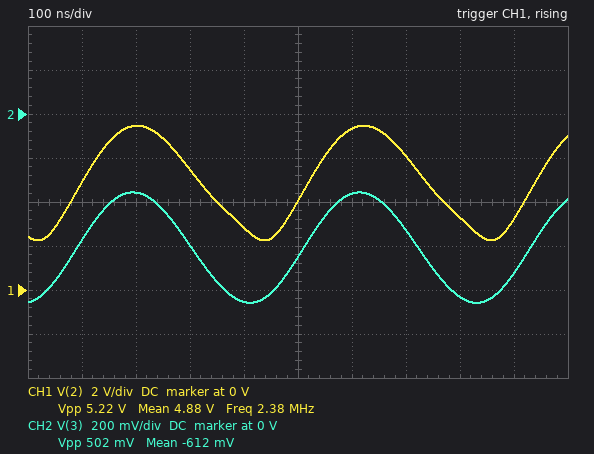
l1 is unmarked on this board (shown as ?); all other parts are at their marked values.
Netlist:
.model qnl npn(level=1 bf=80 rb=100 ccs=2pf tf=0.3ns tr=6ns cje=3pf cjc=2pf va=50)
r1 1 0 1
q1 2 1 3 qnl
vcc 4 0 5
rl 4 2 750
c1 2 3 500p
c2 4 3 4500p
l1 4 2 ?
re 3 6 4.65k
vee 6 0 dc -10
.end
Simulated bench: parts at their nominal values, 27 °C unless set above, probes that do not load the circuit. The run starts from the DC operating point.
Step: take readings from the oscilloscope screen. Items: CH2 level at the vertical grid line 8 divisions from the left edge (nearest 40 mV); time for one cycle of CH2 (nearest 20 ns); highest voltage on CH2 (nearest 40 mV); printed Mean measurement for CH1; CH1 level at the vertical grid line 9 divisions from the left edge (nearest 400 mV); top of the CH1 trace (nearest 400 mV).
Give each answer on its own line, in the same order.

-840 mV
420 ns
-360 mV
4.88 V
3.2 V
7.6 V
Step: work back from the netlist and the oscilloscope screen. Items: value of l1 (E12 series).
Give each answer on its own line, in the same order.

10 µH
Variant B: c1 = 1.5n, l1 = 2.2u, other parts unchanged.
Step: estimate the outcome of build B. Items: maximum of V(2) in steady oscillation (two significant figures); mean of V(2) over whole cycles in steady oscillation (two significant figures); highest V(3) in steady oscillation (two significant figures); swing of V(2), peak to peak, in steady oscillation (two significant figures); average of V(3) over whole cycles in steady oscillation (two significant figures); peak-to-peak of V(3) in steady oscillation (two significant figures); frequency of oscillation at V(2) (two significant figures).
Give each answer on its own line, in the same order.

7.2 V
5.0 V
220 mV
4.4 V
-330 mV
1.1 V
3.2 MHz
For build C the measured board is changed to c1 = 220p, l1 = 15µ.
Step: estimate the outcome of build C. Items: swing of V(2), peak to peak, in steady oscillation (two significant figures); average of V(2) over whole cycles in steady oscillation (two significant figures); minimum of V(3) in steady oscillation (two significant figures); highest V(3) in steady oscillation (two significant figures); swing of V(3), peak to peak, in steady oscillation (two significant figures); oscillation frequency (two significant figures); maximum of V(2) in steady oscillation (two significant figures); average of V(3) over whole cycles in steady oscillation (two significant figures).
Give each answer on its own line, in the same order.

4.8 V
5.0 V
-840 mV
-630 mV
210 mV
2.9 MHz
7.2 V
-730 mV
